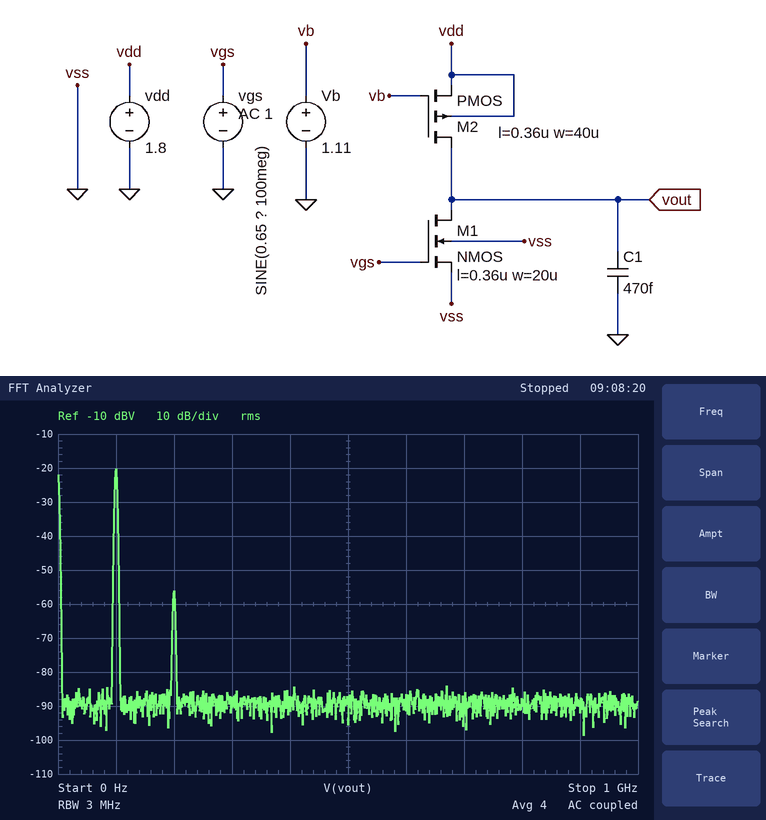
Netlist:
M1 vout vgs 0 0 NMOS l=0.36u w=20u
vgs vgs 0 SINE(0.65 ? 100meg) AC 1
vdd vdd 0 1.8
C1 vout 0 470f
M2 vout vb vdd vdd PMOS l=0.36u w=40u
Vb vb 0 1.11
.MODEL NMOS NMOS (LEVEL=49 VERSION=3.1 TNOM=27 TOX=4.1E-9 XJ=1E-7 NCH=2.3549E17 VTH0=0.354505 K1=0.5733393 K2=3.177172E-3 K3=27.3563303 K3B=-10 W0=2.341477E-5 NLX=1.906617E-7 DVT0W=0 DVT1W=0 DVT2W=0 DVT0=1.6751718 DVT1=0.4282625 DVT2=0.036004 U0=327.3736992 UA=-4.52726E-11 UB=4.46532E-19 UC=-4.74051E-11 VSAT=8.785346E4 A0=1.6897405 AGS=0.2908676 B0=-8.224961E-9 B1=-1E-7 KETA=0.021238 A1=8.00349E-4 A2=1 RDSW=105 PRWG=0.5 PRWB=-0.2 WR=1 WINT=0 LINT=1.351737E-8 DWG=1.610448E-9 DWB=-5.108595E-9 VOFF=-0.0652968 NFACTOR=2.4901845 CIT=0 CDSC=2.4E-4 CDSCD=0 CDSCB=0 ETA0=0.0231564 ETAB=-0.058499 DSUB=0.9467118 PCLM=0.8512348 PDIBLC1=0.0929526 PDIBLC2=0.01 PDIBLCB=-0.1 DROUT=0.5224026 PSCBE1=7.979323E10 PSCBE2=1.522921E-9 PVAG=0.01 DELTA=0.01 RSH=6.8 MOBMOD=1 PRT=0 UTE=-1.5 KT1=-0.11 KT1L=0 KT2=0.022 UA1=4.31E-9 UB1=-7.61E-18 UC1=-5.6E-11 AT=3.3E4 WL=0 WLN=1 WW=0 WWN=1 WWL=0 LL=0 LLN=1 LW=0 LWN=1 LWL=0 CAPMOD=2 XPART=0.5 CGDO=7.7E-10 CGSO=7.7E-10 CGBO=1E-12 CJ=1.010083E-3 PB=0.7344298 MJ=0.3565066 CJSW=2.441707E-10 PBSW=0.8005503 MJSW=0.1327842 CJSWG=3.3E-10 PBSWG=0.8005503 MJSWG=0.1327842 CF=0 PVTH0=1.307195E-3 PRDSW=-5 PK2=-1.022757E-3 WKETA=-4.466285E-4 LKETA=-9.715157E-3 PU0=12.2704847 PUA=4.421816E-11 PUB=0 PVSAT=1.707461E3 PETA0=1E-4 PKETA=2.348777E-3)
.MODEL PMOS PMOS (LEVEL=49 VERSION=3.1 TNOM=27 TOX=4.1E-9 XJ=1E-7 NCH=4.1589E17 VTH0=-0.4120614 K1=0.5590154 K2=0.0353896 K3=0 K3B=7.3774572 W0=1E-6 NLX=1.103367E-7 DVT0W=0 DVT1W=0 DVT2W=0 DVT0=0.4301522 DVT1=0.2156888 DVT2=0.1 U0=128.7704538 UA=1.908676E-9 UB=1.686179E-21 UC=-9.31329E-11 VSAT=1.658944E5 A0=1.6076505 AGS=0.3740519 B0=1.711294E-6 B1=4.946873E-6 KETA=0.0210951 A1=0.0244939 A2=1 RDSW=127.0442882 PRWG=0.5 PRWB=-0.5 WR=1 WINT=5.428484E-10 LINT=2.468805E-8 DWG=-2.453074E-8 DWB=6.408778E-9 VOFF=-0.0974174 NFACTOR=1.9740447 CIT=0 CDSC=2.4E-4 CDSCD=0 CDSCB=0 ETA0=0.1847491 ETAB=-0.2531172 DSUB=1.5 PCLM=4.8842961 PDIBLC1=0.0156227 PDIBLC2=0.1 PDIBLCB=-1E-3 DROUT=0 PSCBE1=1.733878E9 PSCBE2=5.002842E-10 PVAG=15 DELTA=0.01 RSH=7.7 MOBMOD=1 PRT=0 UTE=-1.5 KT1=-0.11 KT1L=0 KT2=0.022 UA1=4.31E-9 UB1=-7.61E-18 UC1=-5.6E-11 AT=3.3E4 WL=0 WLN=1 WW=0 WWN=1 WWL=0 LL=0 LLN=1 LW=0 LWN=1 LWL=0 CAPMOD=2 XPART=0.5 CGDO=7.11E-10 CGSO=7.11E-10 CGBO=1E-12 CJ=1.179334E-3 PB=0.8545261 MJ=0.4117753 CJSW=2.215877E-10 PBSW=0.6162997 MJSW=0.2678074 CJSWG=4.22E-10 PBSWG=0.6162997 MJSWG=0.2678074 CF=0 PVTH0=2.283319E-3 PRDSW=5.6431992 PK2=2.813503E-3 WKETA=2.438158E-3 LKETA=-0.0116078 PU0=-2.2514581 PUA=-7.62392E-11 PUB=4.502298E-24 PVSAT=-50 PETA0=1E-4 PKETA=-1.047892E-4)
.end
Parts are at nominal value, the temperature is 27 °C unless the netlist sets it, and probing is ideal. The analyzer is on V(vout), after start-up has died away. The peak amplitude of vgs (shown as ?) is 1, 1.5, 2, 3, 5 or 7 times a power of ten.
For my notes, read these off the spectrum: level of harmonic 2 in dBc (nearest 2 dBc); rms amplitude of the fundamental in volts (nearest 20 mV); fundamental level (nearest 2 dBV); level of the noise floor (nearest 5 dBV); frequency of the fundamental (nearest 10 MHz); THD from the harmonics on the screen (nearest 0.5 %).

-36 dBc
100 mV
-20 dBV
-90 dBV
100 MHz
1.5 %
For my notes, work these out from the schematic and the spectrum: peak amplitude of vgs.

20 mV
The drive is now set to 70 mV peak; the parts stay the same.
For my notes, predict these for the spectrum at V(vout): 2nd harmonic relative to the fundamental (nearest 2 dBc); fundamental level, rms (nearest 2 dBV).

-22 dBc
-10 dBV
